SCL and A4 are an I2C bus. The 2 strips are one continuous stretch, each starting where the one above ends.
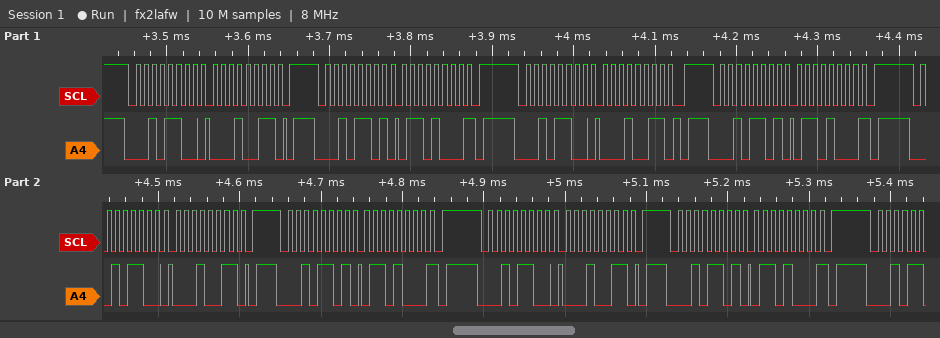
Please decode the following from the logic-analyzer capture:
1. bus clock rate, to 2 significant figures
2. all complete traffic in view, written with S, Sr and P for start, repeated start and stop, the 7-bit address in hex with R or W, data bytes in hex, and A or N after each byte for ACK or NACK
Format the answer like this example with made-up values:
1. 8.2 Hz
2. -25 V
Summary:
1. 100 kHz
2. S 16W A 13 A P S 16R A 68 N P S 16W A 13 A P S 16R A 68 N P S 16W A 13 A P S 16R A 68 N P S 16W A 13 A P S 16R A 68 N P
